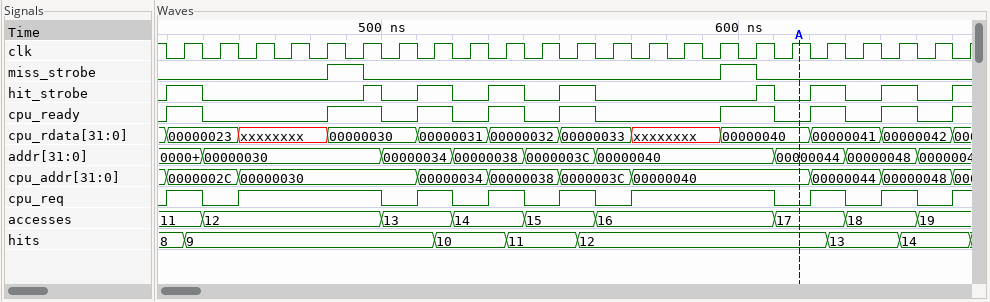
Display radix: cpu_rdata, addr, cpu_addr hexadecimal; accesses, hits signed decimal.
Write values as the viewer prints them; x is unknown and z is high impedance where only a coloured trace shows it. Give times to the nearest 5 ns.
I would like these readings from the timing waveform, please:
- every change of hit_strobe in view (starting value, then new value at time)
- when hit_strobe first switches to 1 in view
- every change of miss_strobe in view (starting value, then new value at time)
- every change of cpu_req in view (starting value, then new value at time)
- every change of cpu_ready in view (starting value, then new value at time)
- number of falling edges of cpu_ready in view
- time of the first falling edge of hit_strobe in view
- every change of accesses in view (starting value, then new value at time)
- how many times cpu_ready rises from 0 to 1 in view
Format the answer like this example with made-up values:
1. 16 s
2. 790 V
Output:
1. 0, 1 at 440 ns, 0 at 450 ns, 1 at 495 ns, 0 at 500 ns, 1 at 510 ns, 0 at 520 ns, 1 at 530 ns, 0 at 540 ns, 1 at 550 ns, 0 at 560 ns, 1 at 605 ns, 0 at 610 ns, 1 at 620 ns, 0 at 630 ns, 1 at 640 ns, 0 at 650 ns, 1 at 660 ns
2. 440 ns
3. 0, 1 at 485 ns, 0 at 495 ns, 1 at 595 ns, 0 at 605 ns
4. 0, 1 at 440 ns, 0 at 450 ns, 1 at 460 ns, 0 at 500 ns, 1 at 510 ns, 0 at 520 ns, 1 at 530 ns, 0 at 540 ns, 1 at 550 ns, 0 at 560 ns, 1 at 570 ns, 0 at 610 ns, 1 at 620 ns, 0 at 630 ns, 1 at 640 ns, 0 at 650 ns, 1 at 660 ns
5. 0, 1 at 440 ns, 0 at 450 ns, 1 at 485 ns, 0 at 500 ns, 1 at 510 ns, 0 at 520 ns, 1 at 530 ns, 0 at 540 ns, 1 at 550 ns, 0 at 560 ns, 1 at 595 ns, 0 at 610 ns, 1 at 620 ns, 0 at 630 ns, 1 at 640 ns, 0 at 650 ns, 1 at 660 ns
6. 8
7. 450 ns
8. 11, 12 at 450 ns, 13 at 500 ns, 14 at 520 ns, 15 at 540 ns, 16 at 560 ns, 17 at 610 ns, 18 at 630 ns, 19 at 650 ns
9. 9
